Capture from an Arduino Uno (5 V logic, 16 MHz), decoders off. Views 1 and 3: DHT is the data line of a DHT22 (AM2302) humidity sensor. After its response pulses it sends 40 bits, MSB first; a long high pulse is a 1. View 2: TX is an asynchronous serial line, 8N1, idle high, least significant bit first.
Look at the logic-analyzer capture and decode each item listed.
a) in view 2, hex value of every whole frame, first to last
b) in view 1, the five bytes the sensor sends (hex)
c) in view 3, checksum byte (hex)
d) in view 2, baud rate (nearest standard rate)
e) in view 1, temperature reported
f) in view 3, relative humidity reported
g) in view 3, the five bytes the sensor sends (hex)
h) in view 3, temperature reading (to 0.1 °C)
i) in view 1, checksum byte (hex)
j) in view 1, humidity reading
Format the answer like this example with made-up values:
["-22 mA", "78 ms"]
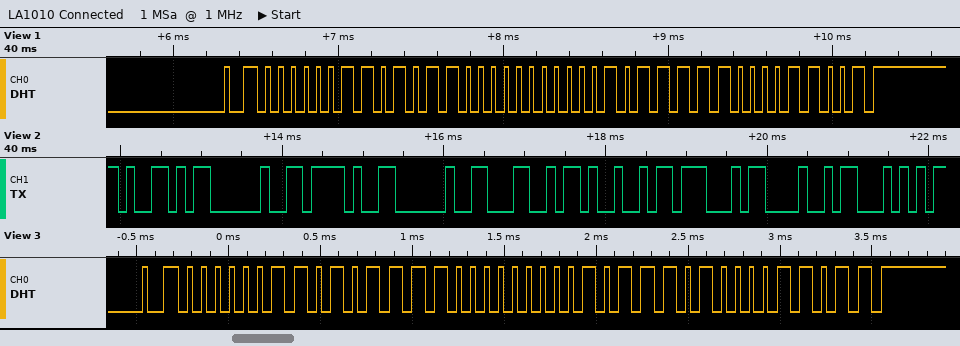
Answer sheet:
["0x59 0x20 0x2F 0x20 0x4C 0x49 0x47 0x48 0x54", "03 58 00 BE 19", "0x1B", "9600 baud", "19.0 °C", "86.2 %", "03 5E 00 BA 1B", "18.6 °C", "0x19", "85.6 %"]
